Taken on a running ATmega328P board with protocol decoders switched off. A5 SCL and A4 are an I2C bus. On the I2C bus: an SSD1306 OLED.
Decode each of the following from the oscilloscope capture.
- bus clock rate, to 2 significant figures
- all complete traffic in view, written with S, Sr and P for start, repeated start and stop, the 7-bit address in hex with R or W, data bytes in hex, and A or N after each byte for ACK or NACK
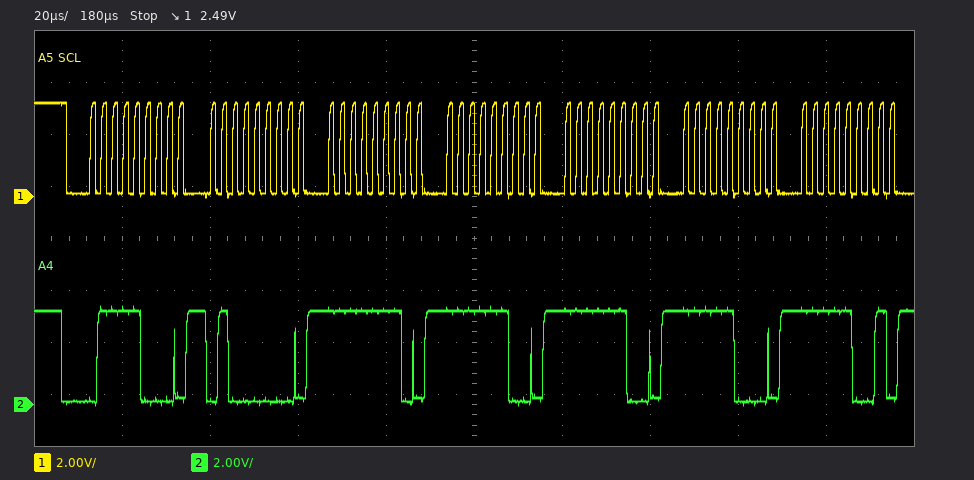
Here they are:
400 kHz
S 3CW A 40 A FE A FC A FC A F8 A F9 A
